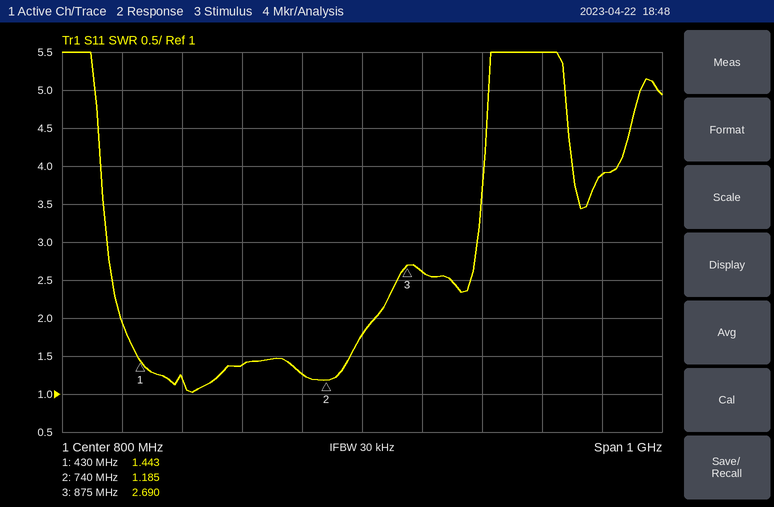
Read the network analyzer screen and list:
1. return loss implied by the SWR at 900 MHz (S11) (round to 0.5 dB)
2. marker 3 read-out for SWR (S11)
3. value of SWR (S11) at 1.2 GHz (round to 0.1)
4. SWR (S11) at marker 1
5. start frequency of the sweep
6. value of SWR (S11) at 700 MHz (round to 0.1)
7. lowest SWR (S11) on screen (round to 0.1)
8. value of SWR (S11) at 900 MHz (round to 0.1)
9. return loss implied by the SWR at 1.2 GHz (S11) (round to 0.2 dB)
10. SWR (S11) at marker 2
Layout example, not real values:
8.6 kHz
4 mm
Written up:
7.0 dB
2.690
3.9
1.443
300 MHz
1.3
1.0
2.6
4.6 dB
1.185
